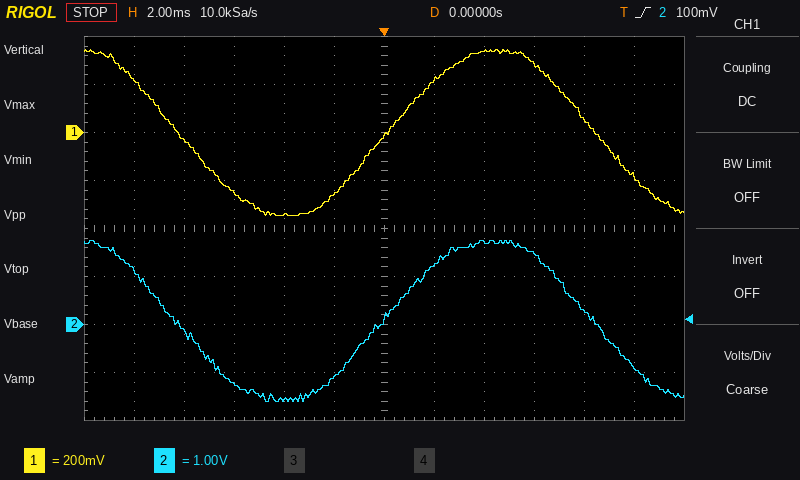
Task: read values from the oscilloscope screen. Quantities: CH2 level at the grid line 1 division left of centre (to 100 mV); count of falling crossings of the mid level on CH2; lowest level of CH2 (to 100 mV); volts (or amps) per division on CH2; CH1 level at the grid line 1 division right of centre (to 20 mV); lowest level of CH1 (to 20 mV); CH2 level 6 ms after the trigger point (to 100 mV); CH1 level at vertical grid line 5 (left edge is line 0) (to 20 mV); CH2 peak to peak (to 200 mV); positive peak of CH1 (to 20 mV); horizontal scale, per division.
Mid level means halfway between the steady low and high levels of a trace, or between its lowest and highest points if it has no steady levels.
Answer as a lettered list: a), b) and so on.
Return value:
a) -1.1 V
b) 2
c) -1.6 V
d) 1 V
e) 220 mV
f) -340 mV
g) 1.5 V
h) -260 mV
i) 3.4 V
j) 340 mV
k) 2 ms
